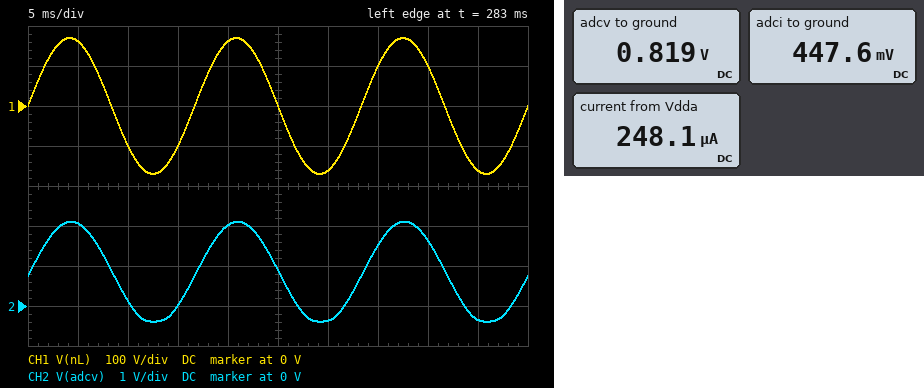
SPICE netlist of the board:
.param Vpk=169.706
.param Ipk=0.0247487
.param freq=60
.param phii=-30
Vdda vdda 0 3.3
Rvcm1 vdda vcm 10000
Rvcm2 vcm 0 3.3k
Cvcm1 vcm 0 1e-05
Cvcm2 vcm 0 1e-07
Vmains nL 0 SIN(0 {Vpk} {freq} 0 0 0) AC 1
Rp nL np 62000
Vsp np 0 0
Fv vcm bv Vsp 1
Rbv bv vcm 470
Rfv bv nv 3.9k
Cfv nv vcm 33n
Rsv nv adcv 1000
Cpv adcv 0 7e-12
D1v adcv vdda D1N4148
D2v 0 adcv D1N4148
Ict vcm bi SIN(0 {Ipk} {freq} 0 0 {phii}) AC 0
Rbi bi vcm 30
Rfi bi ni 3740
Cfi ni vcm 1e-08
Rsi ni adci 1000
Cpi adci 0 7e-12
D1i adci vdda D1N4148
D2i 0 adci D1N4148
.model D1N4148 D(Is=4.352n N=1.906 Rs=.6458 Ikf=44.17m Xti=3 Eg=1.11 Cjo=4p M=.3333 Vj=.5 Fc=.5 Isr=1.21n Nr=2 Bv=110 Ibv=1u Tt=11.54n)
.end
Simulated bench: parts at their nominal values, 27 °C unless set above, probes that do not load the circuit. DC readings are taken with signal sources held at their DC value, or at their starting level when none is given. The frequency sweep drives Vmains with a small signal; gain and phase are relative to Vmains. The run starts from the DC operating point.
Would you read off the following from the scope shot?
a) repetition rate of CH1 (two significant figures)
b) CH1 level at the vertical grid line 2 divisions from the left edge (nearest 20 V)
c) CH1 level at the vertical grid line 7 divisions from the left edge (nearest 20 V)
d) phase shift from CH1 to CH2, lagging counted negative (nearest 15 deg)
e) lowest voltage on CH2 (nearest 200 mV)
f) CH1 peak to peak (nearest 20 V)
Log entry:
60 Hz
-100 V
100 V
0 deg
-400 mV
340 V
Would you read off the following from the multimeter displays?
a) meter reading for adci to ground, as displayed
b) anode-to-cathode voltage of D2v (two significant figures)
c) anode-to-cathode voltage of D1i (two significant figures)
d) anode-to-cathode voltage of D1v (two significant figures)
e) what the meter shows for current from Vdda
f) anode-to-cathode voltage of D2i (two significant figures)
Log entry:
447.6 mV
-820 mV
-2.9 V
-2.5 V
248.1 µA
-450 mV
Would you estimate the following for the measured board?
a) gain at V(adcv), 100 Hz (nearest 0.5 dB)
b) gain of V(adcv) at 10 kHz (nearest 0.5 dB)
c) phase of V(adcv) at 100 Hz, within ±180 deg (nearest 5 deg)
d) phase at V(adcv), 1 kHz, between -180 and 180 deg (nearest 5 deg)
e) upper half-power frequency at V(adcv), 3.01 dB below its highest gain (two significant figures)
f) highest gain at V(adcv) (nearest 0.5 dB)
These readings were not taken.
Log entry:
-42.5 dB
-61.5 dB
-5 deg
-40 deg
1.1 kHz
-42.5 dB
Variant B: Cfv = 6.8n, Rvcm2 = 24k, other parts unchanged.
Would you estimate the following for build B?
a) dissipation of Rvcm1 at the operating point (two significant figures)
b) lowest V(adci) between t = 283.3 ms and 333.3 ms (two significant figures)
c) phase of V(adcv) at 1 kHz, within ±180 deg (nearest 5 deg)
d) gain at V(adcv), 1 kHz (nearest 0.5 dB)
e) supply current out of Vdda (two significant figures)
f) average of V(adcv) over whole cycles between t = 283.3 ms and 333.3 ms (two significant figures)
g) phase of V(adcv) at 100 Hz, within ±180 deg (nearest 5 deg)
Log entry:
94 µW
1.6 V
-10 deg
-42.5 dB
97 µA
2.3 V
0 deg
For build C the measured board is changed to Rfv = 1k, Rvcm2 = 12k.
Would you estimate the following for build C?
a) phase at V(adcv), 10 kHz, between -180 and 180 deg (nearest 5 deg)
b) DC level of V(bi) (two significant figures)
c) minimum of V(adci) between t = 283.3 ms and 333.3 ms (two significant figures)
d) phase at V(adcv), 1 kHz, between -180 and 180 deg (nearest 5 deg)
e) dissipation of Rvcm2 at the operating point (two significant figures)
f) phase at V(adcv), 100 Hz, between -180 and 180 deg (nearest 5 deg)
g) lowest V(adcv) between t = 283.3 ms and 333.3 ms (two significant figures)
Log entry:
-70 deg
1.4 V
1.1 V
-15 deg
270 µW
0 deg
510 mV
